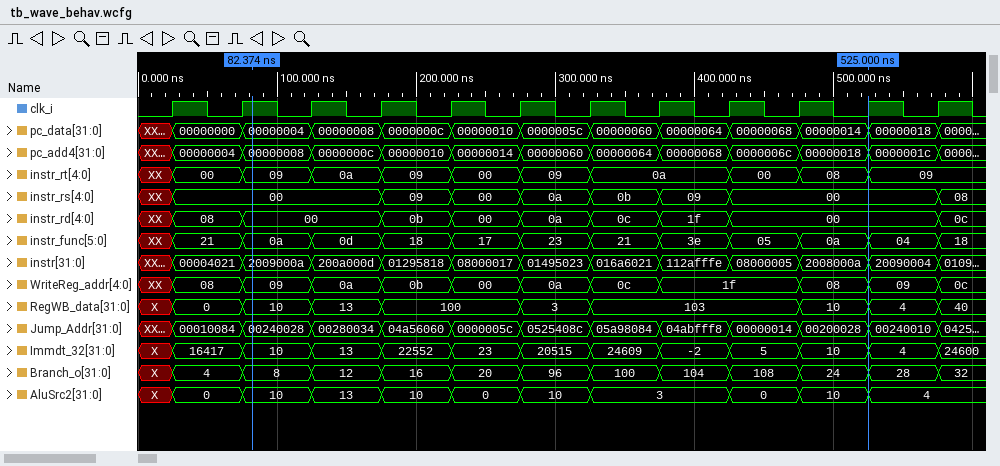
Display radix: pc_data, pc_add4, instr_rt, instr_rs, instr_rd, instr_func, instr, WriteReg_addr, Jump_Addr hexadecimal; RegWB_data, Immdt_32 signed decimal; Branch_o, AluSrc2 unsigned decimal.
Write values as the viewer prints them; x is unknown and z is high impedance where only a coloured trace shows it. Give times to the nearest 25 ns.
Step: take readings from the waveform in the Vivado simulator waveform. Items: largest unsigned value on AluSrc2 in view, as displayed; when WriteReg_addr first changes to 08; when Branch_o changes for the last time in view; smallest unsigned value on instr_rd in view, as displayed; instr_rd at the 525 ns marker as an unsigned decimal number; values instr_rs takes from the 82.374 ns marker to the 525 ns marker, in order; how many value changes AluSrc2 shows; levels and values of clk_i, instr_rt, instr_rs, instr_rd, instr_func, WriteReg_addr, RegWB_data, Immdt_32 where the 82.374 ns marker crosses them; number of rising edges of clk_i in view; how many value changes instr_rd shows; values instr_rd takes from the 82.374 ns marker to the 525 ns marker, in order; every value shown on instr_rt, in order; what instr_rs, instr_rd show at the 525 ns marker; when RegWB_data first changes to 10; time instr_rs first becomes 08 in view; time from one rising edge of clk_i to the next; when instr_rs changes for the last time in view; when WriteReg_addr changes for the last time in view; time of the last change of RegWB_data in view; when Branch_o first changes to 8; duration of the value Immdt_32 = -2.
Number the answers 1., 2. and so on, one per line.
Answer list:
1. 13
2. 25 ns
3. 575 ns
4. 00
5. 0
6. 00, 09, 00, 0a, 0b, 09, 00
7. 10
8. clk_i=1, instr_rt=09, instr_rs=00, instr_rd=00, instr_func=0a, WriteReg_addr=09, RegWB_data=10, Immdt_32=10
9. 12
10. 9
11. 00, 0b, 00, 0a, 0c, 1f, 00
12. XX, 00, 09, 0a, 09, 00, 09, 0a, 00, 08, 09
13. instr_rs=00, instr_rd=00
14. 75 ns
15. 575 ns
16. 50 ns
17. 575 ns
18. 575 ns
19. 575 ns
20. 75 ns
21. 50 ns
